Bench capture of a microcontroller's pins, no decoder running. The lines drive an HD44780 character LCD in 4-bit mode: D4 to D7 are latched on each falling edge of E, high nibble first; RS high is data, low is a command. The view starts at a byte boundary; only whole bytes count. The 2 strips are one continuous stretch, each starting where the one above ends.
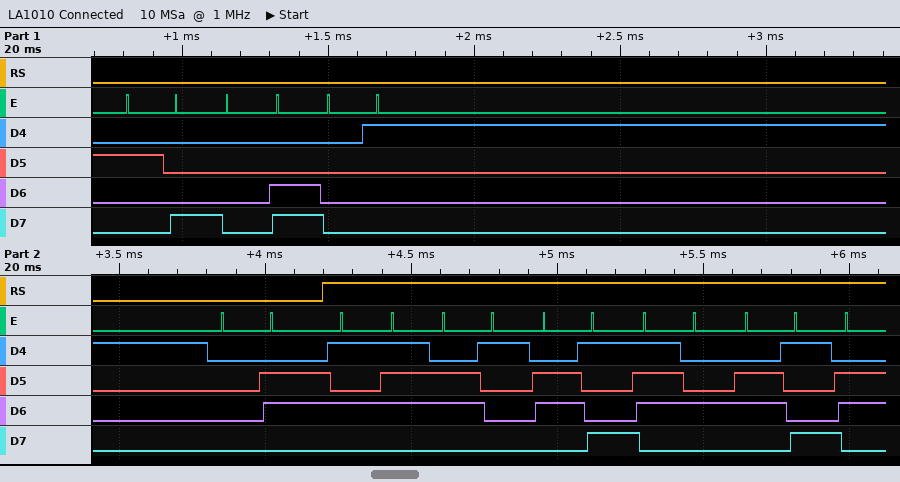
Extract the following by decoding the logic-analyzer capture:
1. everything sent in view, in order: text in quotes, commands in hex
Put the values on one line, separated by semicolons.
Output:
0x28 0x0C 0x01 0x06 "Waiti"
